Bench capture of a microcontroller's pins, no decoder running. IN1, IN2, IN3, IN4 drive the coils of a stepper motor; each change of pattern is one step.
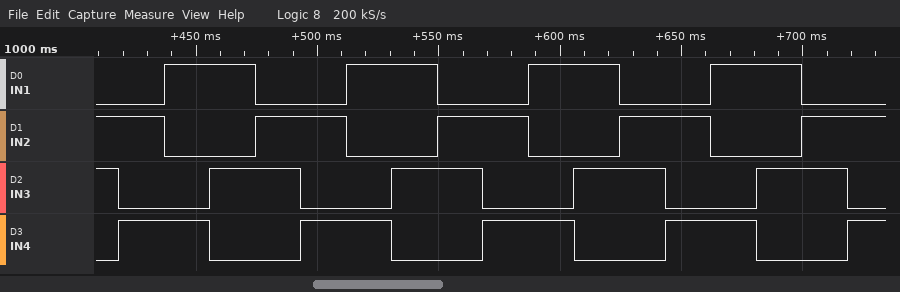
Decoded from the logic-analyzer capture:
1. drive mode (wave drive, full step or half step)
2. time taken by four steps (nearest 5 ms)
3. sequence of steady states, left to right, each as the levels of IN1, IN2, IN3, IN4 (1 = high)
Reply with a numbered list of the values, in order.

1. full step
2. 75 ms
3. 0110 0101 1001 1010 0110 0101 1001 1010 0110 0101 1001 1010 0110 0101 1001 1010 0110 0101
